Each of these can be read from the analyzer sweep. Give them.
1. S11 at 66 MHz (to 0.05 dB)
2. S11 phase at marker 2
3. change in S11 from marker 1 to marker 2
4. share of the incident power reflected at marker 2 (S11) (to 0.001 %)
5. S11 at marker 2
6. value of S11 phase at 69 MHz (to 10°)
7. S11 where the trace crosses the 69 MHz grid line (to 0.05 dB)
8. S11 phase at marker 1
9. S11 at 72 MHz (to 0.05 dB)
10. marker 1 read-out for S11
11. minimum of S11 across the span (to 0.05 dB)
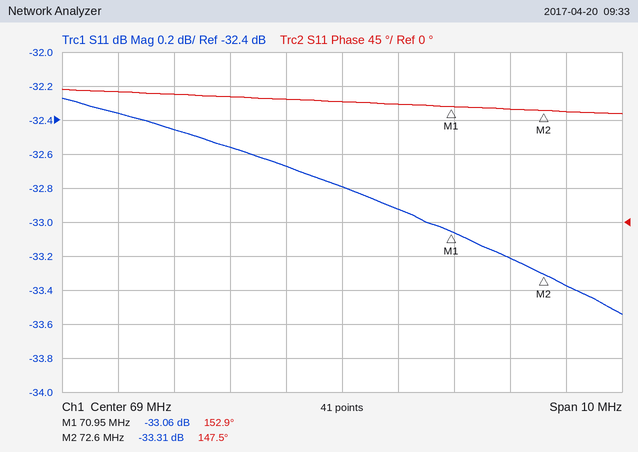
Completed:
-32.45 dB
147.5°
-0.25 dB
0.047 %
-33.31 dB
160°
-32.80 dB
152.9°
-33.20 dB
-33.06 dB
-33.55 dB
